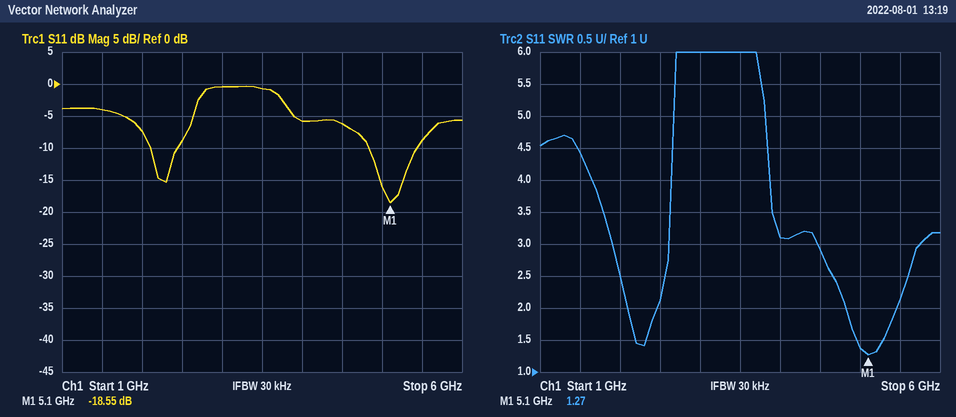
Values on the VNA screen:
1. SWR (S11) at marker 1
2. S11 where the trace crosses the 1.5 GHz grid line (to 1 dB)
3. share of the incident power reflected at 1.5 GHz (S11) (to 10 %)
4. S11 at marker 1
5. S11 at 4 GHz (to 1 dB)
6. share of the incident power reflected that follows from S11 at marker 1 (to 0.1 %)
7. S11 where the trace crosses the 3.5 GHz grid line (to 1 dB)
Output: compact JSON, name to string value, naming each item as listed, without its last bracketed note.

{"SWR (S11) at marker 1": "1.27", "S11 where the trace crosses the 1.5 GHz grid line": "-4 dB", "share of the incident power reflected at 1.5 GHz (S11)": "40 %", "S11 at marker 1": "-18.55 dB", "S11 at 4 GHz": "-6 dB", "share of the incident power reflected that follows from S11 at marker 1": "1.4 %", "S11 where the trace crosses the 3.5 GHz grid line": "-1 dB"}
